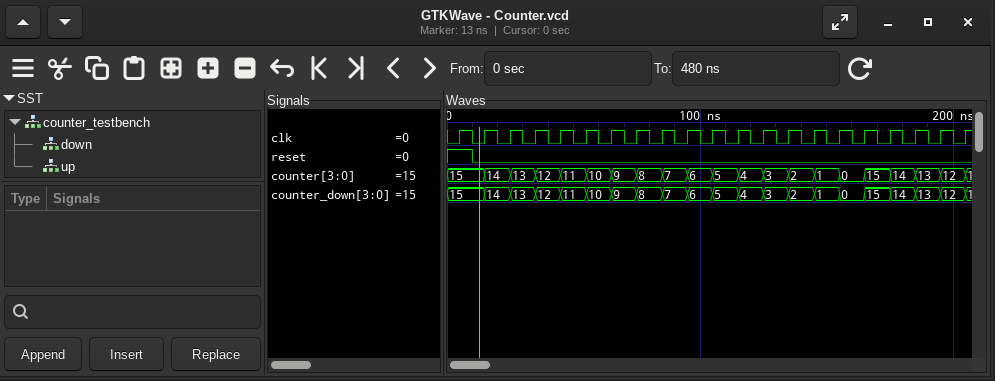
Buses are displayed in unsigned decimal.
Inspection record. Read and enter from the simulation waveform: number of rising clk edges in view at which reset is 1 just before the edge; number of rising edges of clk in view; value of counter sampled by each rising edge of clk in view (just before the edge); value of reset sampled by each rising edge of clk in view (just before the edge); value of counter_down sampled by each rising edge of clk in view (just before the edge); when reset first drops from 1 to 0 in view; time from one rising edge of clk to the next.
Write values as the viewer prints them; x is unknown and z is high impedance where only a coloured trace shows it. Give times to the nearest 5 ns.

1
21
15, 15, 14, 13, 12, 11, 10, 9, 8, 7, 6, 5, 4, 3, 2, 1, 0, 15, 14, 13, 12
1 0 0 0 0 0 0 0 0 0 0 0 0 0 0 0 0 0 0 0 0
15, 15, 14, 13, 12, 11, 10, 9, 8, 7, 6, 5, 4, 3, 2, 1, 0, 15, 14, 13, 12
10 ns
10 ns
